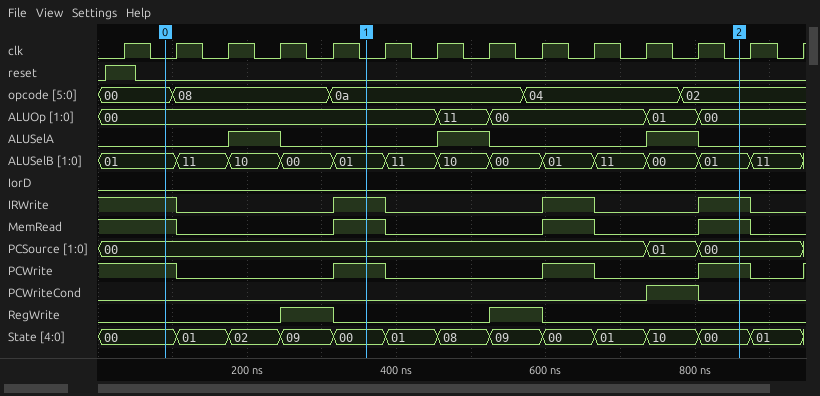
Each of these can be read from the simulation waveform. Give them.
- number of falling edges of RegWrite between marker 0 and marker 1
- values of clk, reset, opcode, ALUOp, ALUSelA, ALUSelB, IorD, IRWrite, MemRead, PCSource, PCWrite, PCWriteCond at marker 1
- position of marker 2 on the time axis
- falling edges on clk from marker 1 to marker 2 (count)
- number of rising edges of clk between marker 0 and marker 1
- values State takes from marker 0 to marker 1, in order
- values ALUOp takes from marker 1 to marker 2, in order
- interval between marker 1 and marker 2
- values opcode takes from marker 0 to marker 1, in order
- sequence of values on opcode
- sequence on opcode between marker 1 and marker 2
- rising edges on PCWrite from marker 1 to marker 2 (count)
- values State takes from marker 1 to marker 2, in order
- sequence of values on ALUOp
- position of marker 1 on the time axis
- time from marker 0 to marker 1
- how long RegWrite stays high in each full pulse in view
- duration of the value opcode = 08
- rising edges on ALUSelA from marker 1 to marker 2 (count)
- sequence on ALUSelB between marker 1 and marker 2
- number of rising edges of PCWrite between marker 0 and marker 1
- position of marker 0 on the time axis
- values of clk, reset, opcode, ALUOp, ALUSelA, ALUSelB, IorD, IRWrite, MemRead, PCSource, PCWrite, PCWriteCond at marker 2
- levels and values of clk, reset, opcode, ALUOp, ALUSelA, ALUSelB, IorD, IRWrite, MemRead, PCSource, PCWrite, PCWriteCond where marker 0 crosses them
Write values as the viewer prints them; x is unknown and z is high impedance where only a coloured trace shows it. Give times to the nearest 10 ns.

1
clk=0, reset=0, opcode=0a, ALUOp=00, ALUSelA=0, ALUSelB=01, IorD=0, IRWrite=1, MemRead=1, PCSource=00, PCWrite=1, PCWriteCond=0
860 ns
7
4
00, 01, 02, 09, 00
00, 11, 00, 01, 00
500 ns
00, 08, 0a
00, 08, 0a, 04, 02
0a, 04, 02
2
00, 01, 08, 09, 00, 01, 10, 00
00, 11, 00, 01, 00
360 ns
270 ns
70 ns, 70 ns
210 ns
2
01, 11, 10, 00, 01, 11, 00, 01
1
90 ns
clk=0, reset=0, opcode=02, ALUOp=00, ALUSelA=0, ALUSelB=01, IorD=0, IRWrite=1, MemRead=1, PCSource=00, PCWrite=1, PCWriteCond=0
clk=0, reset=0, opcode=00, ALUOp=00, ALUSelA=0, ALUSelB=01, IorD=0, IRWrite=1, MemRead=1, PCSource=00, PCWrite=1, PCWriteCond=0
